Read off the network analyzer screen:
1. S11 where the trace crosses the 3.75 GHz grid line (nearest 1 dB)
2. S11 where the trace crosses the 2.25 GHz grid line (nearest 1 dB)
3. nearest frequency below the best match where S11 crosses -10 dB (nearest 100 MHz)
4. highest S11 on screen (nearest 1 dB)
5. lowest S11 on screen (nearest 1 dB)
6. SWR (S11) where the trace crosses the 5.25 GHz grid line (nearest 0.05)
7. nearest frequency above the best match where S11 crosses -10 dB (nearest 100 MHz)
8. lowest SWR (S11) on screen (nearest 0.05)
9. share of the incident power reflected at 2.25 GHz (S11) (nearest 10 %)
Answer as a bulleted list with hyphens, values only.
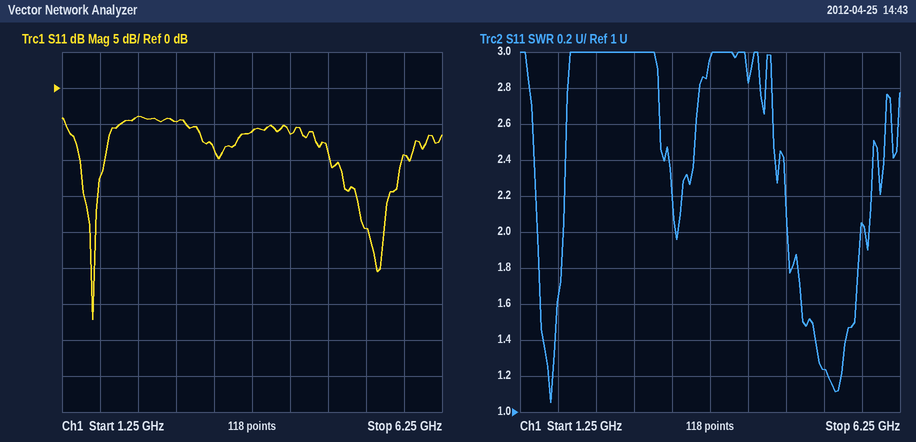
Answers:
- -6 dB
- -4 dB
- 1.5 GHz
- -4 dB
- -32 dB
- 1.25
- 1.8 GHz
- 1.05
- 40 %
